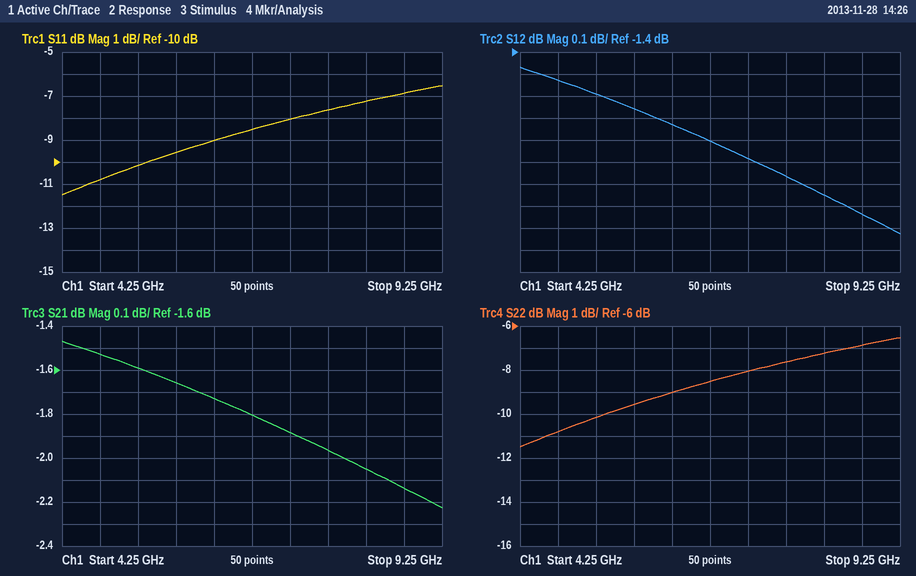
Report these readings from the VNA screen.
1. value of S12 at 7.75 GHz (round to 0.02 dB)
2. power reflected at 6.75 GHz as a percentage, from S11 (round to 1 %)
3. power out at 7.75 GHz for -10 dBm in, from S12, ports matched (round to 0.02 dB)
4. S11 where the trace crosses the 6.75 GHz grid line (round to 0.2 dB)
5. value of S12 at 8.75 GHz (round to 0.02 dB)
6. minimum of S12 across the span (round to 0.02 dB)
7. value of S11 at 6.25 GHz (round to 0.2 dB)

-1.96 dB
14 %
-11.96 dBm
-8.6 dB
-2.14 dB
-2.22 dB
-9.0 dB
